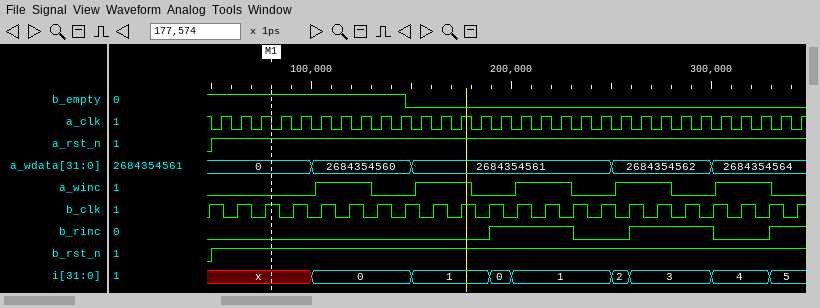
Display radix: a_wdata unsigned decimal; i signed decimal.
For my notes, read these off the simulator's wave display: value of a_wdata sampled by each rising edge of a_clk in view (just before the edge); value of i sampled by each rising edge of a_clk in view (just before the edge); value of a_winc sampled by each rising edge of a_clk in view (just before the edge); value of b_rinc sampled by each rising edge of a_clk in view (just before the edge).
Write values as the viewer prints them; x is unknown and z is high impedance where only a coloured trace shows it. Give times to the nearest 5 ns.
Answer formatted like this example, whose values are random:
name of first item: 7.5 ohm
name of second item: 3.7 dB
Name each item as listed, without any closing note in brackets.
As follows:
value of a_wdata sampled by each rising edge of a_clk in view: 0, 0, 0, 0, 0, 2684354560, 2684354560, 2684354560, 2684354560, 2684354560, 2684354561, 2684354561, 2684354561, 2684354561, 2684354561, 2684354561, 2684354561, 2684354561, 2684354561, 2684354561, 2684354562, 2684354562, 2684354562, 2684354562, 2684354562, 2684354564, 2684354564, 2684354564, 2684354564, 2684354564
value of i sampled by each rising edge of a_clk in view: x, x, x, x, x, 0, 0, 0, 0, 0, 1, 1, 1, 1, 0, 1, 1, 1, 1, 1, 2, 3, 3, 3, 3, 4, 4, 4, 5, 5
value of a_winc sampled by each rising edge of a_clk in view: 0 0 0 0 0 1 1 1 0 0 1 1 1 0 0 1 1 1 0 0 1 1 1 0 0 1 1 1 0 0
value of b_rinc sampled by each rising edge of a_clk in view: 0 0 0 0 0 0 0 0 0 0 0 0 0 0 1 1 1 1 0 0 0 1 1 1 1 0 0 0 1 1
